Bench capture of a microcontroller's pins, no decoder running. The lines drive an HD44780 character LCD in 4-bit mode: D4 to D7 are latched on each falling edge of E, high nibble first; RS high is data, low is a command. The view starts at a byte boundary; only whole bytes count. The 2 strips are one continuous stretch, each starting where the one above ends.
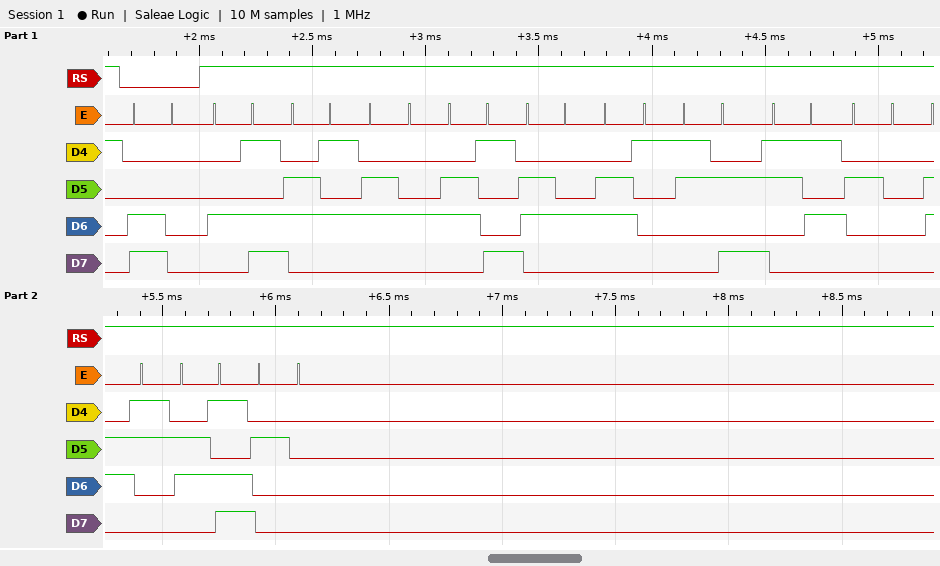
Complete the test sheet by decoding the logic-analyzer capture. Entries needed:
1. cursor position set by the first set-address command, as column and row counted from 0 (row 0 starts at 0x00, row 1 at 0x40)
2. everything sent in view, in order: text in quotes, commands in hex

column 0, row 1
0xC0 "Medida:5 cm "
